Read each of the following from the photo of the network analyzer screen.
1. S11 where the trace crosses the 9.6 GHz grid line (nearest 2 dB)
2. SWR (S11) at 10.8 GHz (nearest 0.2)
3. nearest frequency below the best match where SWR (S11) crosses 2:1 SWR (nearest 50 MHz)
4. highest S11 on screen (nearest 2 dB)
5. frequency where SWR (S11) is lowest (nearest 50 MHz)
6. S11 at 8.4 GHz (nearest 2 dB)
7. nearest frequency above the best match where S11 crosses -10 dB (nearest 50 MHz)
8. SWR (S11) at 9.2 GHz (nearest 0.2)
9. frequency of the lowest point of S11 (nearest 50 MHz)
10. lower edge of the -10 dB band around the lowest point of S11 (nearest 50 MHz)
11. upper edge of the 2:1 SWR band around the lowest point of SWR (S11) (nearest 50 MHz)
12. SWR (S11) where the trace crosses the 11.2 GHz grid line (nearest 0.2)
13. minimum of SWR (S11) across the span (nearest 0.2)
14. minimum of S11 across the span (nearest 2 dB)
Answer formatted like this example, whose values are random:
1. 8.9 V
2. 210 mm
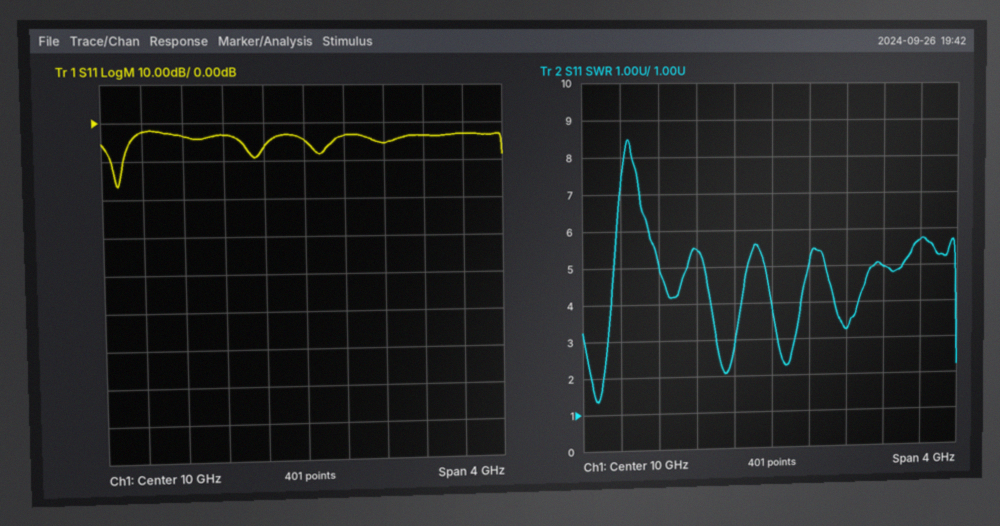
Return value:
1. -6 dB
2. 3.2
3. 8.10 GHz
4. -2 dB
5. 8.15 GHz
6. -2 dB
7. 8.20 GHz
8. 5.4
9. 8.15 GHz
10. 8.10 GHz
11. 8.20 GHz
12. 5.0
13. 1.4
14. -16 dB
